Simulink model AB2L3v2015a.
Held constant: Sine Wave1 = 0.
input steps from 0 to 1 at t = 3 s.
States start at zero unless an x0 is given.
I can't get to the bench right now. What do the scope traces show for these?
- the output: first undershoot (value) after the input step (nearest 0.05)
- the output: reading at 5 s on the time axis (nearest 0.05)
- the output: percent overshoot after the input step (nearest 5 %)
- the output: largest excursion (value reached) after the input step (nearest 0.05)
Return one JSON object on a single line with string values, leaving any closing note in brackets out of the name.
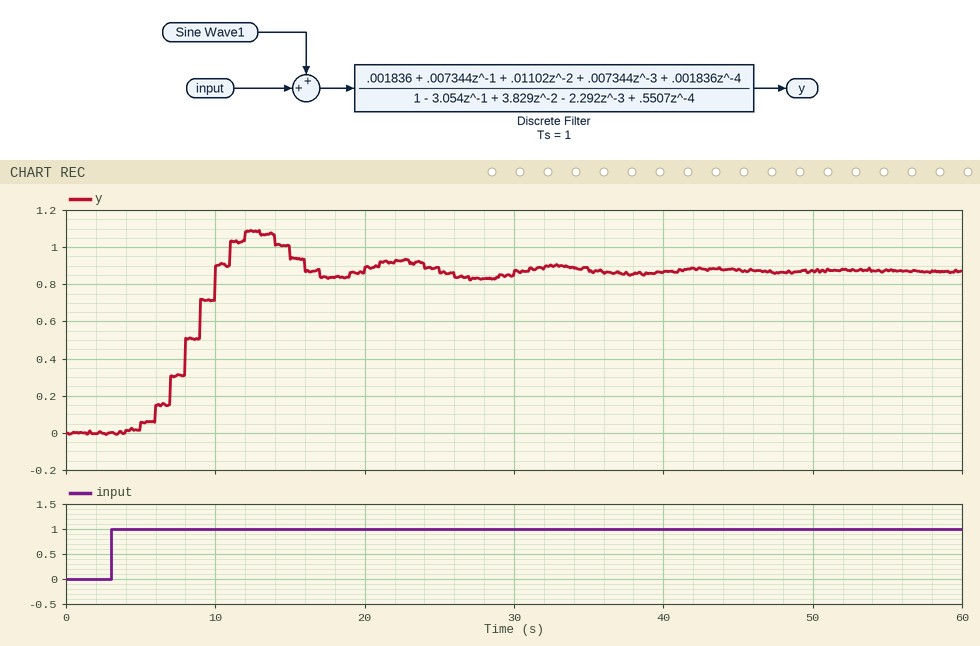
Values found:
{"the output: first undershoot (value) after the input step": "0.85", "the output: reading at 5 s on the time axis": "0.05", "the output: percent overshoot after the input step": "25 %", "the output: largest excursion (value reached) after the input step": "1.10"}
